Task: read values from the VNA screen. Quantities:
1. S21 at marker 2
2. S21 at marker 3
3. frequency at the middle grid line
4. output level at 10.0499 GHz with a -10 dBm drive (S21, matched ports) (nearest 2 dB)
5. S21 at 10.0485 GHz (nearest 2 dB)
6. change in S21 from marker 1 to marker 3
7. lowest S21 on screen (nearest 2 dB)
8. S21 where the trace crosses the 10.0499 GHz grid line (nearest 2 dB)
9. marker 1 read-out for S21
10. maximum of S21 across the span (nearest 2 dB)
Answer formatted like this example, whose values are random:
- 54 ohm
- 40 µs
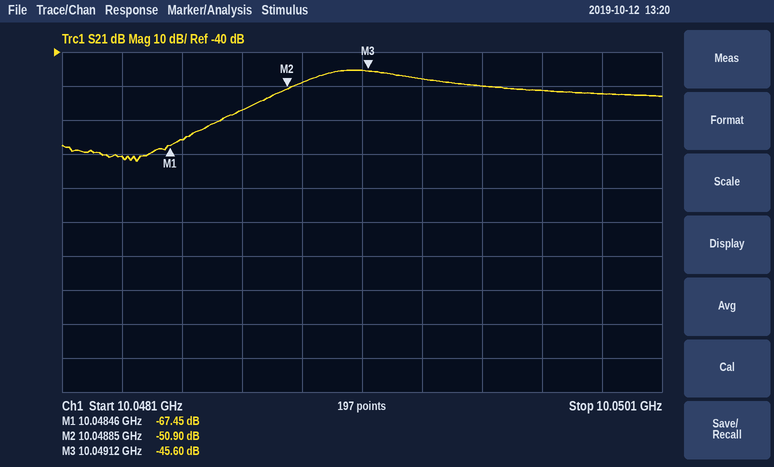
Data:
- -50.90 dB
- -45.60 dB
- 10.0491 GHz
- -62 dBm
- -66 dB
- 21.85 dB
- -72 dB
- -52 dB
- -67.45 dB
- -46 dB
